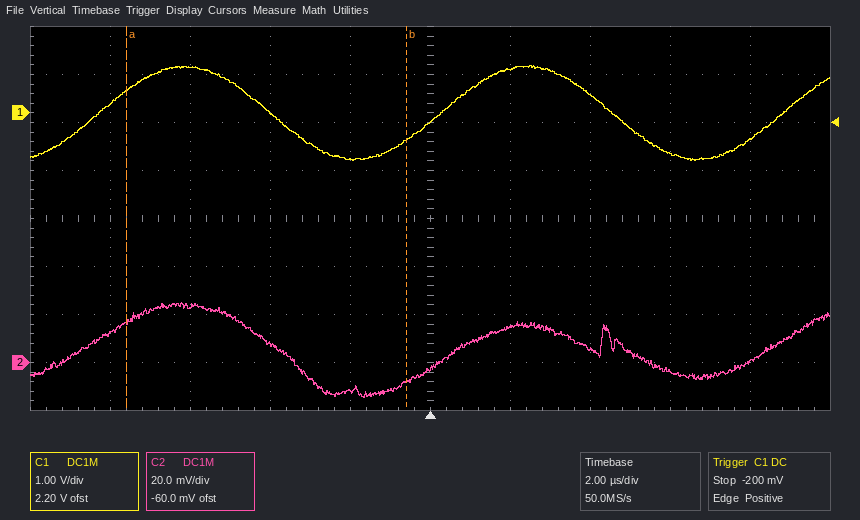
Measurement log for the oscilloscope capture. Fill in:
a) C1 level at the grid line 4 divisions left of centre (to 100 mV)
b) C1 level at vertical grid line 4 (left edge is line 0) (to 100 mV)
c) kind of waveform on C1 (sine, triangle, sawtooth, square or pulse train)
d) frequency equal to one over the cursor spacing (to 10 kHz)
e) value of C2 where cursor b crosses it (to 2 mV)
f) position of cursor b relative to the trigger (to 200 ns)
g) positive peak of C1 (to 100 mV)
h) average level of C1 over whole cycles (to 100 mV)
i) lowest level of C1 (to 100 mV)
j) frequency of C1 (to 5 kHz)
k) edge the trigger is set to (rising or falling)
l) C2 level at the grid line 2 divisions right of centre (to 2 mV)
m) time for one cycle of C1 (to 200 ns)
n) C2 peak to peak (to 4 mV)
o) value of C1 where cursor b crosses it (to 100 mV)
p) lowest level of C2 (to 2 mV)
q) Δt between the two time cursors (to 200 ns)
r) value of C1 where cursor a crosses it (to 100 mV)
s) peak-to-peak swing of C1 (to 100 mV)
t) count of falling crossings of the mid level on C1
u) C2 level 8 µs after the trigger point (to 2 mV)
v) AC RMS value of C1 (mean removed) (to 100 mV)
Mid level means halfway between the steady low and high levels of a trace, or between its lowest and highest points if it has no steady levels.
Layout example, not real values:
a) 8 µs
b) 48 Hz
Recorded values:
a) 200 mV
b) -1.0 V
c) sine
d) 140 kHz
e) -8 mV
f) -600 ns
g) 1.0 V
h) 0.0 V
i) -1.0 V
j) 115 kHz
k) rising
l) 6 mV
m) 8.6 µs
n) 40 mV
o) -600 mV
p) -14 mV
q) 7.0 µs
r) 500 mV
s) 2.0 V
t) 2
u) 0 mV
v) 700 mV
